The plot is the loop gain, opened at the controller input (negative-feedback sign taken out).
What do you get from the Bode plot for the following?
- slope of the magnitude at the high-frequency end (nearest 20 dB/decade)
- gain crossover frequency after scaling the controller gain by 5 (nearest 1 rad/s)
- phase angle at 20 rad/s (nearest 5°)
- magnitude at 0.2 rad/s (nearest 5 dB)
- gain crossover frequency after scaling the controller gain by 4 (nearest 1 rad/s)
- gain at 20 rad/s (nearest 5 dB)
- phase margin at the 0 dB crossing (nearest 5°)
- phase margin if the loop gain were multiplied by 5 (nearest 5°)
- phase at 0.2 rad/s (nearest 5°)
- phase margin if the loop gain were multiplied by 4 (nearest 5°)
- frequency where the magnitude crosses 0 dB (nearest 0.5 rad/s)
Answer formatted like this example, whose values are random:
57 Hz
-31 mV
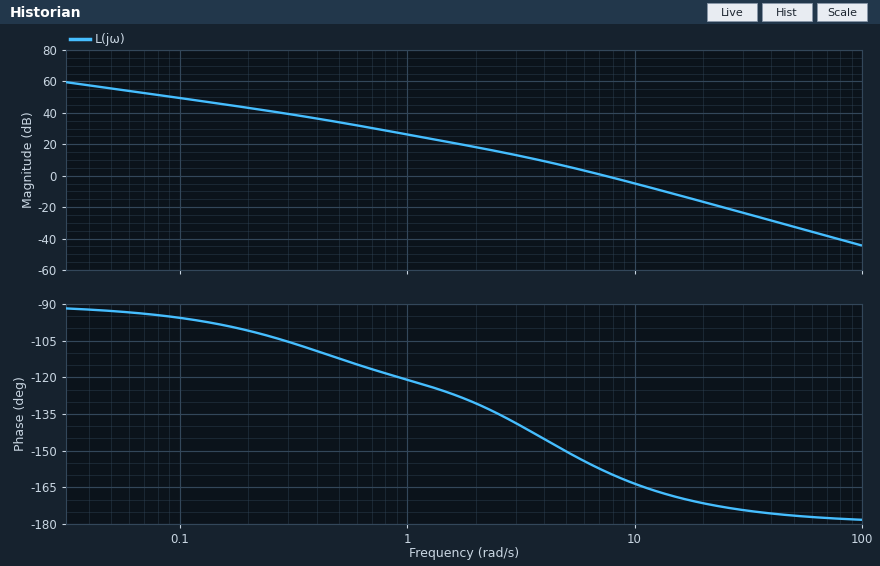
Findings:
-40 dB/decade
17 rad/s
-170°
45 dB
15 rad/s
-15 dB
20°
10°
-100°
10°
7.5 rad/s
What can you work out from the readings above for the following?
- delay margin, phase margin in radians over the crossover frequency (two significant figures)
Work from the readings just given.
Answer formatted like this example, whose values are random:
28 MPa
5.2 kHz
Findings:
0.047 s
